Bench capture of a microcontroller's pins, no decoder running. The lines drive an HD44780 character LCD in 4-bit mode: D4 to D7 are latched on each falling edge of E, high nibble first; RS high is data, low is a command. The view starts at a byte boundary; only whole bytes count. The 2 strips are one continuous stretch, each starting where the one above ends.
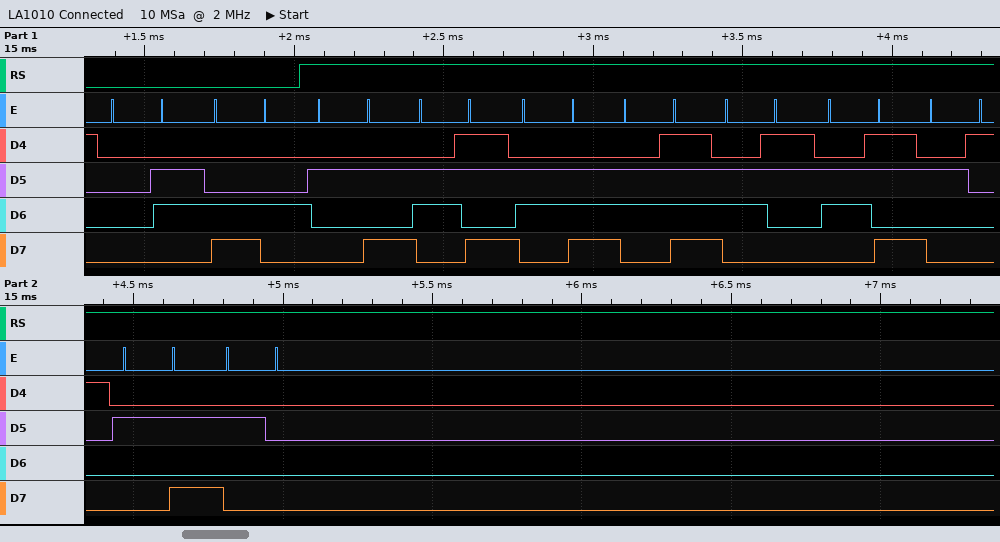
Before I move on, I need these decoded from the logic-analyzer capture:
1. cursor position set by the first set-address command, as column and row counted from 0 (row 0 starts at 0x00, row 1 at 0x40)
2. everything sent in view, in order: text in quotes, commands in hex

column 4, row 1
0x06 0xC4 "*knock!* "
